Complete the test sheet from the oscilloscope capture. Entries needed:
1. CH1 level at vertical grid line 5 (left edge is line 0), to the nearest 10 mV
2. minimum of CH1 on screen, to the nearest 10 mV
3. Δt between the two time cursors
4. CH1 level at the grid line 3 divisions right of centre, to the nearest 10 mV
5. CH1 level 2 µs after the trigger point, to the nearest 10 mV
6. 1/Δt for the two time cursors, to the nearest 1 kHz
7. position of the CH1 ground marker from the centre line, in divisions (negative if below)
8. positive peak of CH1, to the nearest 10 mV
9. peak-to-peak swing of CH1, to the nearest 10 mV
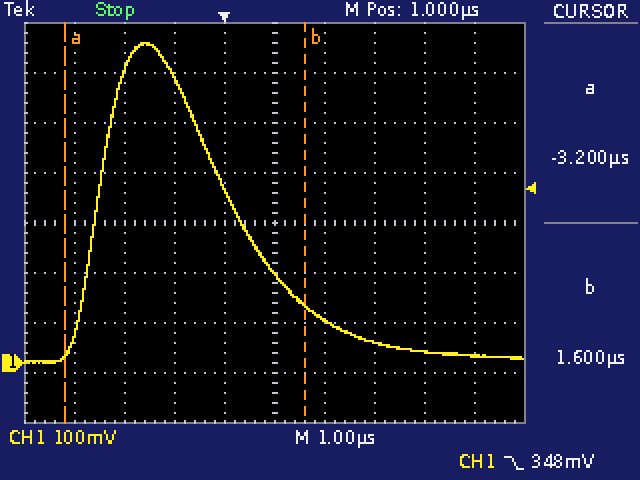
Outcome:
180 mV
0 mV
4.8 µs
20 mV
90 mV
208 kHz
-2.8 div
640 mV
640 mV
